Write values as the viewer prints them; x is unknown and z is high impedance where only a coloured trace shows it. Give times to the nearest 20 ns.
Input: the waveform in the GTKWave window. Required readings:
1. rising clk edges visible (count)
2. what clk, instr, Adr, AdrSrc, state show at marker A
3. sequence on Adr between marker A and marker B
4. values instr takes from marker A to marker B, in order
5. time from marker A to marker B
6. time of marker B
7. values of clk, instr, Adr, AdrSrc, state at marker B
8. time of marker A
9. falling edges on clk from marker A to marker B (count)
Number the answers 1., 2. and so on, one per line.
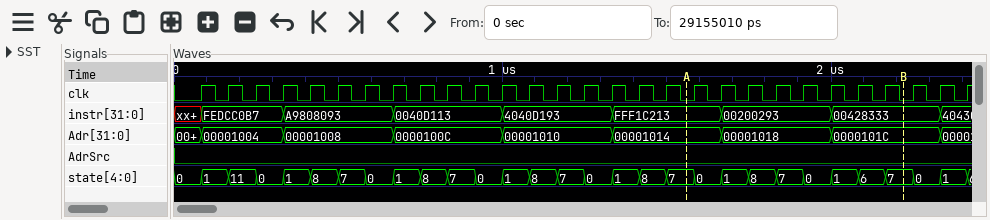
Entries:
1. 29
2. clk=0, instr=FFF1C213, Adr=00001014, AdrSrc=0, state=7
3. 00001014, 00001018, 0000101C
4. FFF1C213, 00200293, 00428333
5. 660 ns
6. 2220 ns
7. clk=0, instr=00428333, Adr=0000101C, AdrSrc=0, state=7
8. 1560 ns
9. 8
